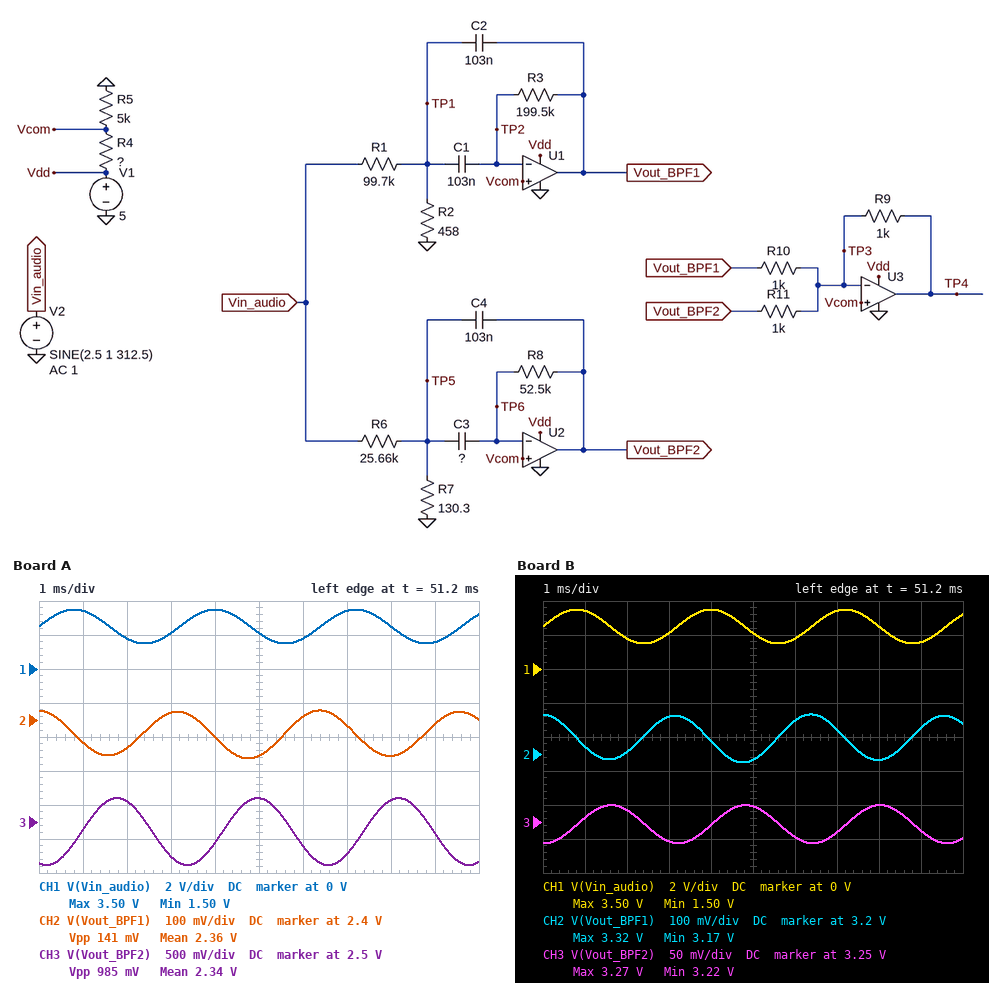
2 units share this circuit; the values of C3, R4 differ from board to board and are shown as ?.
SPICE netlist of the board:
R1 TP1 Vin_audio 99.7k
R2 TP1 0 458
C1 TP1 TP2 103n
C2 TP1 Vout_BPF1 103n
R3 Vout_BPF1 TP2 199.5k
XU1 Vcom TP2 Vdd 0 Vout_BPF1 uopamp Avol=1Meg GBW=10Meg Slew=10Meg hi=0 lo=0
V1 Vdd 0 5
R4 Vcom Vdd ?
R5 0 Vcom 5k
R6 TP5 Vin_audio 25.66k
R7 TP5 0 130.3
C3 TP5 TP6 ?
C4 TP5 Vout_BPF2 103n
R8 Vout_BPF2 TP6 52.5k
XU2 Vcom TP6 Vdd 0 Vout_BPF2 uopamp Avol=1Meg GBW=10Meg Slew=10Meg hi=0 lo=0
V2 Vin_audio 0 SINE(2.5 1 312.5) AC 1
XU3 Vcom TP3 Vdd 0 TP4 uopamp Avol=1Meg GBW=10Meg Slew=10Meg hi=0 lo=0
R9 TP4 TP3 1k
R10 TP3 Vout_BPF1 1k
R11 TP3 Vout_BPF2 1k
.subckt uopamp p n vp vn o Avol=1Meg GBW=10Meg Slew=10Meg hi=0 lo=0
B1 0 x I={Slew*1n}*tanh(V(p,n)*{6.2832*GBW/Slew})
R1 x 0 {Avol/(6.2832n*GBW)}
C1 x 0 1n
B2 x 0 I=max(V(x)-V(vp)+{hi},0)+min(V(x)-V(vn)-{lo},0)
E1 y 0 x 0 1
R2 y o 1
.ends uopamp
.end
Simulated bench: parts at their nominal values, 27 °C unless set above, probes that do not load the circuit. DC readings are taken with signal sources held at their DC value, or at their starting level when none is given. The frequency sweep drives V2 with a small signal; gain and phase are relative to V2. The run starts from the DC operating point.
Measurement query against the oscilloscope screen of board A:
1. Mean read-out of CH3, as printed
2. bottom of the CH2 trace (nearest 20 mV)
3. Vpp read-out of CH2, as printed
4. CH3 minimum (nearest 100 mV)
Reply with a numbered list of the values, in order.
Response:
1. 2.34 V
2. 2.28 V
3. 141 mV
4. 1.9 V
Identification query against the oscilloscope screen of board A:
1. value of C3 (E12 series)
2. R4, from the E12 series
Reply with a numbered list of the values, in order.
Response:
1. 270 nF
2. 5.6 kΩ
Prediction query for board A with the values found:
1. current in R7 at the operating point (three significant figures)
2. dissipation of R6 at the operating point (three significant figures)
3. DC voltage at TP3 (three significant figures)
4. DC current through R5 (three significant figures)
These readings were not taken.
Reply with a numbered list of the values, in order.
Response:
1. 96.9 µA
2. 241 µW
3. 2.36 V
4. 472 µA
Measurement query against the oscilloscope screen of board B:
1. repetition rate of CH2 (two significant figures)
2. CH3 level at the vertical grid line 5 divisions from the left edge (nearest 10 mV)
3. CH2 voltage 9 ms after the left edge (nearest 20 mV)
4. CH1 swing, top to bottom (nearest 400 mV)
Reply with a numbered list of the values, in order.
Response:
1. 310 Hz
2. 3.27 V
3. 3.28 V
4. 2.0 V
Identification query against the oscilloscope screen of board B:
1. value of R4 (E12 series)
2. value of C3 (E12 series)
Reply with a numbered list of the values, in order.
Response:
1. 2.7 kΩ
2. 47 nF
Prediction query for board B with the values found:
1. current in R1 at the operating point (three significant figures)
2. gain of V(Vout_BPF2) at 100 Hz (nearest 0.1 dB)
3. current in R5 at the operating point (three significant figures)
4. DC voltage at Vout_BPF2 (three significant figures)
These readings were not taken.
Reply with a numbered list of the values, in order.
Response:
1. 25.0 µA
2. -42.0 dB
3. 649 µA
4. 3.25 V
